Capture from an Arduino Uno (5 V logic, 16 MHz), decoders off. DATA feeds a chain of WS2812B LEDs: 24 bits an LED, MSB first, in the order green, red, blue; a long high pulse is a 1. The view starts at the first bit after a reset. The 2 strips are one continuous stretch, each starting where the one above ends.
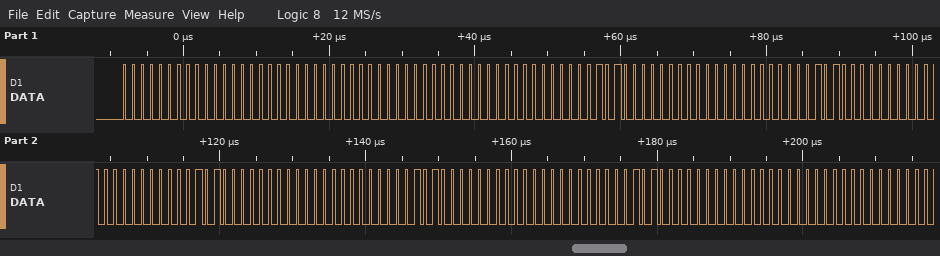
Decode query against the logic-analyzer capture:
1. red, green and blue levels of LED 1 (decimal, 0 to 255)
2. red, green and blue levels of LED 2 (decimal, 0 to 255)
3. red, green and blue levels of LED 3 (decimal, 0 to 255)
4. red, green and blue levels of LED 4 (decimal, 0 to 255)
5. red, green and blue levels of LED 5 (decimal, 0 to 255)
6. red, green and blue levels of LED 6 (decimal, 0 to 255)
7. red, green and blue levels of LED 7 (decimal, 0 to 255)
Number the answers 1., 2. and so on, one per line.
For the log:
1. 0, 0, 0
2. 0, 0, 0
3. 0, 10, 0
4. 0, 10, 0
5. 0, 10, 0
6. 0, 10, 0
7. 0, 10, 0
